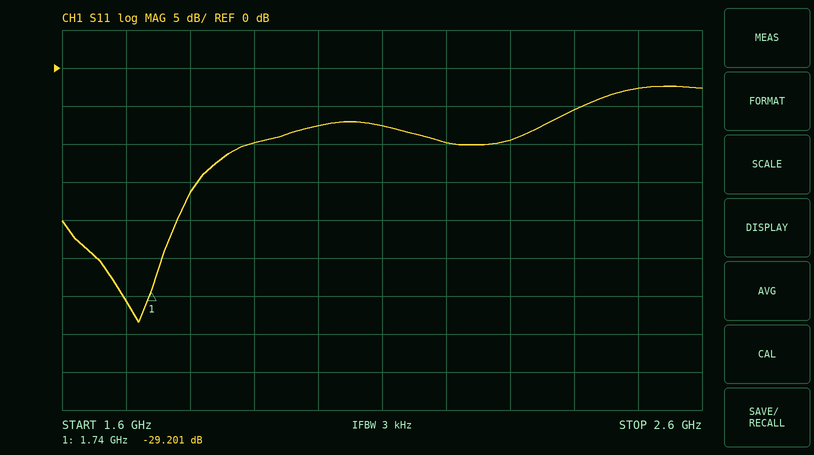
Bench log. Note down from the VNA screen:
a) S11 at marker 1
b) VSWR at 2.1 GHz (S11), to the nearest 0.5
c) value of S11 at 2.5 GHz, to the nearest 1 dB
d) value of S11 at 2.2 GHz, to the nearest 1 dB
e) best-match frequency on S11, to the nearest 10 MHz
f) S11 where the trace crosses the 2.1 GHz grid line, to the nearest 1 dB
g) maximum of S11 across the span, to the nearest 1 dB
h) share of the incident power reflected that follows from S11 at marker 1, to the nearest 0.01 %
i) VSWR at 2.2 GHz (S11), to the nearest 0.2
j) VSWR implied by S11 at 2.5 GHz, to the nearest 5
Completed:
-29.201 dB
2.5
-3 dB
-10 dB
1.72 GHz
-8 dB
-2 dB
0.12 %
2.0
5
